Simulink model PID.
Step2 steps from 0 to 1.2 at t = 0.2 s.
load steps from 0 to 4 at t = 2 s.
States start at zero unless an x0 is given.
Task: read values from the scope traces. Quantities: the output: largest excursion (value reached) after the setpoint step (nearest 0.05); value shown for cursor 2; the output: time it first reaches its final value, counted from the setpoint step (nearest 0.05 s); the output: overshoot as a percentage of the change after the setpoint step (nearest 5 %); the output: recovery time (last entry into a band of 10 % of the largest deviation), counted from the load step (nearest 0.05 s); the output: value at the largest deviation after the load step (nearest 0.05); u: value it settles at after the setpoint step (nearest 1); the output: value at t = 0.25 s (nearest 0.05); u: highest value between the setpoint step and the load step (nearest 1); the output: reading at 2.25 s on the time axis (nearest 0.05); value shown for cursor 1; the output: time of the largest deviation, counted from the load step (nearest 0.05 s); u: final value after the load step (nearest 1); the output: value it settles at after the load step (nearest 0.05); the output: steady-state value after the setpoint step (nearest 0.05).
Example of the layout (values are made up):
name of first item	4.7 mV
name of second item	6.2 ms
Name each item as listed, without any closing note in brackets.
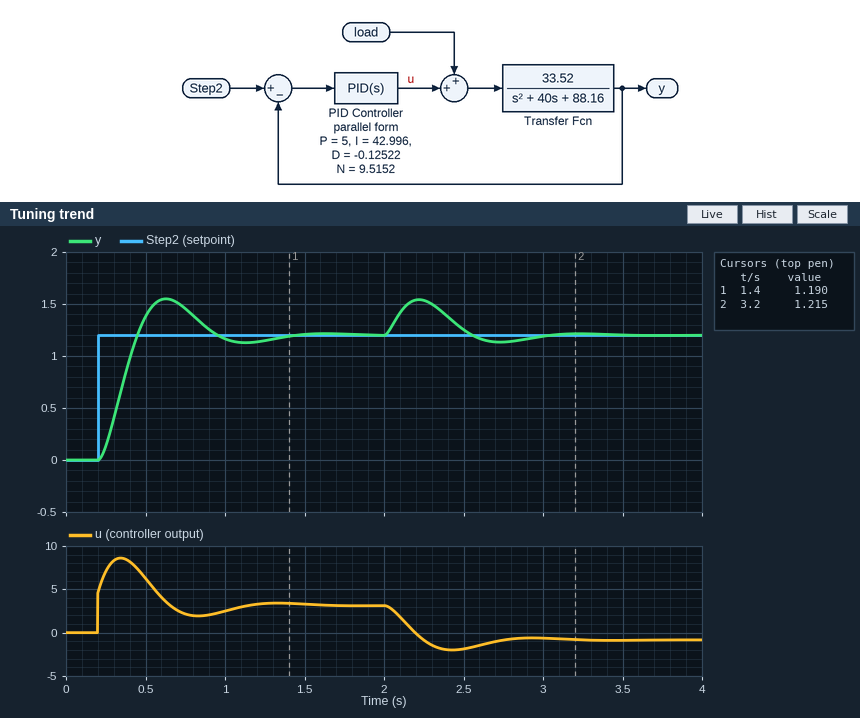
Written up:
the output: largest excursion (value reached) after the setpoint step	1.55
value shown for cursor 2	1.215
the output: time it first reaches its final value, counted from the setpoint step	0.25 s
the output: overshoot as a percentage of the change after the setpoint step	30 %
the output: recovery time (last entry into a band of 10 % of the largest deviation), counted from the load step	0.90 s
the output: value at the largest deviation after the load step	1.55
u: value it settles at after the setpoint step	3
the output: value at t = 0.25 s	0.15
u: highest value between the setpoint step and the load step	9
the output: reading at 2.25 s on the time axis	1.55
value shown for cursor 1	1.190
the output: time of the largest deviation, counted from the load step	0.20 s
u: final value after the load step	-1
the output: value it settles at after the load step	1.20
the output: steady-state value after the setpoint step	1.20
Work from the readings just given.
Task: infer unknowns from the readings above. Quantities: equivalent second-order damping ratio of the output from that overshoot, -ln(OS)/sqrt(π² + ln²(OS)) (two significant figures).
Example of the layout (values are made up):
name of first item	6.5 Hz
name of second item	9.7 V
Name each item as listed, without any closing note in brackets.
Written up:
equivalent second-order damping ratio of the output from that overshoot, -ln(OS)/sqrt(π² + ln²(OS))	0.36
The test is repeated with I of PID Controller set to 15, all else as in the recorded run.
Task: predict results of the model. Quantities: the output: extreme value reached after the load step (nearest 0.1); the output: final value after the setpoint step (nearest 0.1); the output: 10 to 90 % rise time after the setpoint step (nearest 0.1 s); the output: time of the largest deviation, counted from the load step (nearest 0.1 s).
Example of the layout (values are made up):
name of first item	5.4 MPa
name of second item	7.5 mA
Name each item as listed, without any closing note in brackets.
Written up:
the output: extreme value reached after the load step	1.6
the output: final value after the setpoint step	1.2
the output: 10 to 90 % rise time after the setpoint step	0.3 s
the output: time of the largest deviation, counted from the load step	0.3 s
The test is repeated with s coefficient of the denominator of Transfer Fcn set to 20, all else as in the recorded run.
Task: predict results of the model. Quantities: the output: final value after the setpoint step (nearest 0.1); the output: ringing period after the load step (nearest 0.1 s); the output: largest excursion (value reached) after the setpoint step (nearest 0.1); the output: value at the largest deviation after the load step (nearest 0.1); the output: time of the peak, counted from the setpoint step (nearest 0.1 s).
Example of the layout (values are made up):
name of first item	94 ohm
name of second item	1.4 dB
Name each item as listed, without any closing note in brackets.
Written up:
the output: final value after the setpoint step	1.2
the output: ringing period after the load step	0.6 s
the output: largest excursion (value reached) after the setpoint step	1.6
the output: value at the largest deviation after the load step	1.7
the output: time of the peak, counted from the setpoint step	0.3 s
